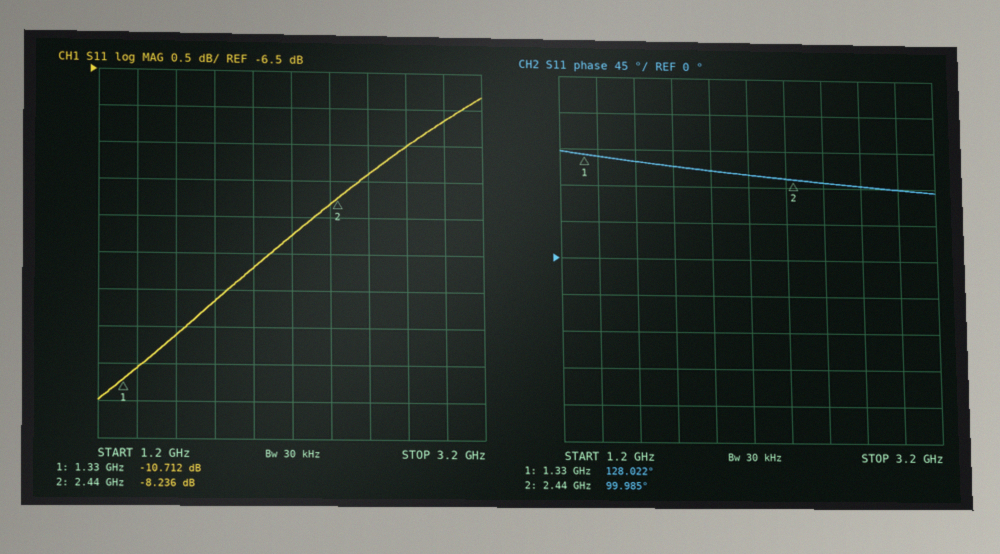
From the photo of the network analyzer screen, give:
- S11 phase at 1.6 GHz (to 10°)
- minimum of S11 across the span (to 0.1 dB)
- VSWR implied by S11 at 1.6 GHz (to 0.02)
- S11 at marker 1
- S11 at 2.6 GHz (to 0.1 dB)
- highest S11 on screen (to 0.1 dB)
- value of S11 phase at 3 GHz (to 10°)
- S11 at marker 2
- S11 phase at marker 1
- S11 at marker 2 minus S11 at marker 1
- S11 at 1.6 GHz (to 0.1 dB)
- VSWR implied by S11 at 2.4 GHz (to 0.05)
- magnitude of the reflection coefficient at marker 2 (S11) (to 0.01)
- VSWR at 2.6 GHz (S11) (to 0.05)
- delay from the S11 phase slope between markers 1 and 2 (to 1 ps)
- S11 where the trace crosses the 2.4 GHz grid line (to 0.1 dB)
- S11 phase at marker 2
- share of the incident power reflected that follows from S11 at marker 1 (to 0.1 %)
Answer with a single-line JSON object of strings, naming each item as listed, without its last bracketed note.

{"S11 phase at 1.6 GHz": "120°", "minimum of S11 across the span": "-11.0 dB", "VSWR implied by S11 at 1.6 GHz": "1.90", "S11 at marker 1": "-10.712 dB", "S11 at 2.6 GHz": "-7.9 dB", "highest S11 on screen": "-6.8 dB", "value of S11 phase at 3 GHz": "90°", "S11 at marker 2": "-8.236 dB", "S11 phase at marker 1": "128.022°", "S11 at marker 2 minus S11 at marker 1": "2.476 dB", "S11 at 1.6 GHz": "-10.1 dB", "VSWR implied by S11 at 2.4 GHz": "2.25", "magnitude of the reflection coefficient at marker 2 (S11)": "0.39", "VSWR at 2.6 GHz (S11)": "2.35", "delay from the S11 phase slope between markers 1 and 2": "70 ps", "S11 where the trace crosses the 2.4 GHz grid line": "-8.3 dB", "S11 phase at marker 2": "99.985°", "share of the incident power reflected that follows from S11 at marker 1": "8.5 %"}
